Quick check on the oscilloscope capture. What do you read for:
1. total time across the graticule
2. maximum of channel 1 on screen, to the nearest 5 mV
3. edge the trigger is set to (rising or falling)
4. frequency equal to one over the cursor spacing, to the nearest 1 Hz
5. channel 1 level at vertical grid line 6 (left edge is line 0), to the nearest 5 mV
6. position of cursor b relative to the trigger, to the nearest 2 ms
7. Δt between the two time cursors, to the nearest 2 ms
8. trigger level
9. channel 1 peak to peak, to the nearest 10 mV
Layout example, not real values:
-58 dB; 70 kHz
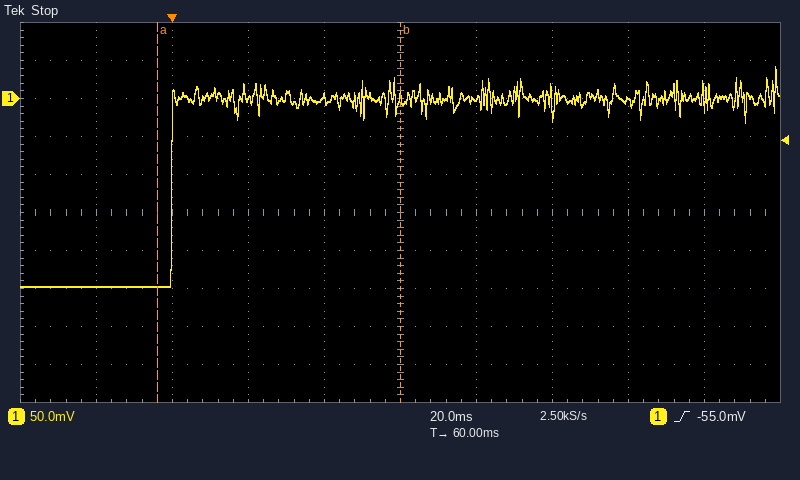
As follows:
200 ms; 40 mV; rising; 16 Hz; 0 mV; +60 ms; 64 ms; -55.0 mV; 290 mV
